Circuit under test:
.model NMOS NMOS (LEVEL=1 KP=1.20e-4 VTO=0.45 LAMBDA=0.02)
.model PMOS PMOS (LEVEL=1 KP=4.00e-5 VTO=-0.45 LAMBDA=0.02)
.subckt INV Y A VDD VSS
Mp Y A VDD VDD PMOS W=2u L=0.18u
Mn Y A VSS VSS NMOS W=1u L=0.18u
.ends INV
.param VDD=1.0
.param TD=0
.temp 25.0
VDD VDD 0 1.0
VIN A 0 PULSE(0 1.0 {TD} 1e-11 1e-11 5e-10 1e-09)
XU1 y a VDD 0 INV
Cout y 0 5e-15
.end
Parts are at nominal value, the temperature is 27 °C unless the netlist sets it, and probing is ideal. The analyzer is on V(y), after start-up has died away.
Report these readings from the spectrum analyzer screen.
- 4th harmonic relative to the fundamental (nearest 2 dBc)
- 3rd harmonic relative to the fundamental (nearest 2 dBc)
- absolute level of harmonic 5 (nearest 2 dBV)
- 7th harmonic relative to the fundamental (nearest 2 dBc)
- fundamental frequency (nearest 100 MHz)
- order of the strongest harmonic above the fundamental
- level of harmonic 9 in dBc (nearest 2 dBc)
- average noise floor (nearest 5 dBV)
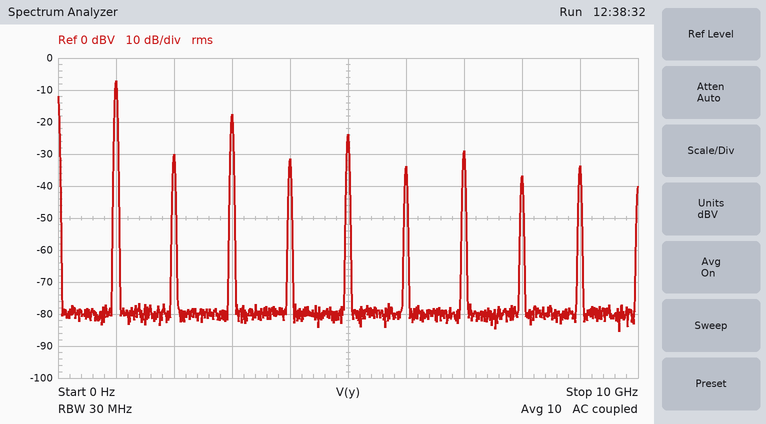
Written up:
-24 dBc
-10 dBc
-24 dBV
-22 dBc
1.0 GHz
3
-26 dBc
-80 dBV
